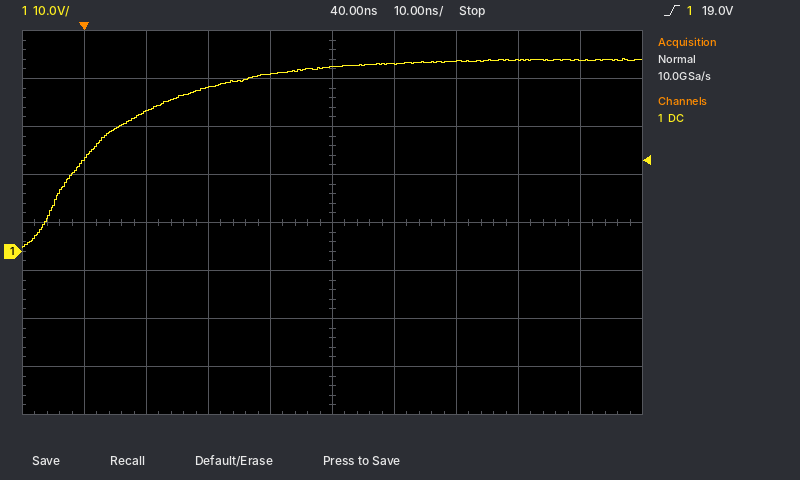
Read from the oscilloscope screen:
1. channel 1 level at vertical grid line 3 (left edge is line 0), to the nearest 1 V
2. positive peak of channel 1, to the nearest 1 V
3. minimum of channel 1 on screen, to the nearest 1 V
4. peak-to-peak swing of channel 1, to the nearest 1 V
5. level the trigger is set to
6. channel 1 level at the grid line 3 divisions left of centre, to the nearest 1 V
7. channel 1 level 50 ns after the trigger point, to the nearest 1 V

34 V
40 V
1 V
39 V
19.0 V
29 V
39 V
